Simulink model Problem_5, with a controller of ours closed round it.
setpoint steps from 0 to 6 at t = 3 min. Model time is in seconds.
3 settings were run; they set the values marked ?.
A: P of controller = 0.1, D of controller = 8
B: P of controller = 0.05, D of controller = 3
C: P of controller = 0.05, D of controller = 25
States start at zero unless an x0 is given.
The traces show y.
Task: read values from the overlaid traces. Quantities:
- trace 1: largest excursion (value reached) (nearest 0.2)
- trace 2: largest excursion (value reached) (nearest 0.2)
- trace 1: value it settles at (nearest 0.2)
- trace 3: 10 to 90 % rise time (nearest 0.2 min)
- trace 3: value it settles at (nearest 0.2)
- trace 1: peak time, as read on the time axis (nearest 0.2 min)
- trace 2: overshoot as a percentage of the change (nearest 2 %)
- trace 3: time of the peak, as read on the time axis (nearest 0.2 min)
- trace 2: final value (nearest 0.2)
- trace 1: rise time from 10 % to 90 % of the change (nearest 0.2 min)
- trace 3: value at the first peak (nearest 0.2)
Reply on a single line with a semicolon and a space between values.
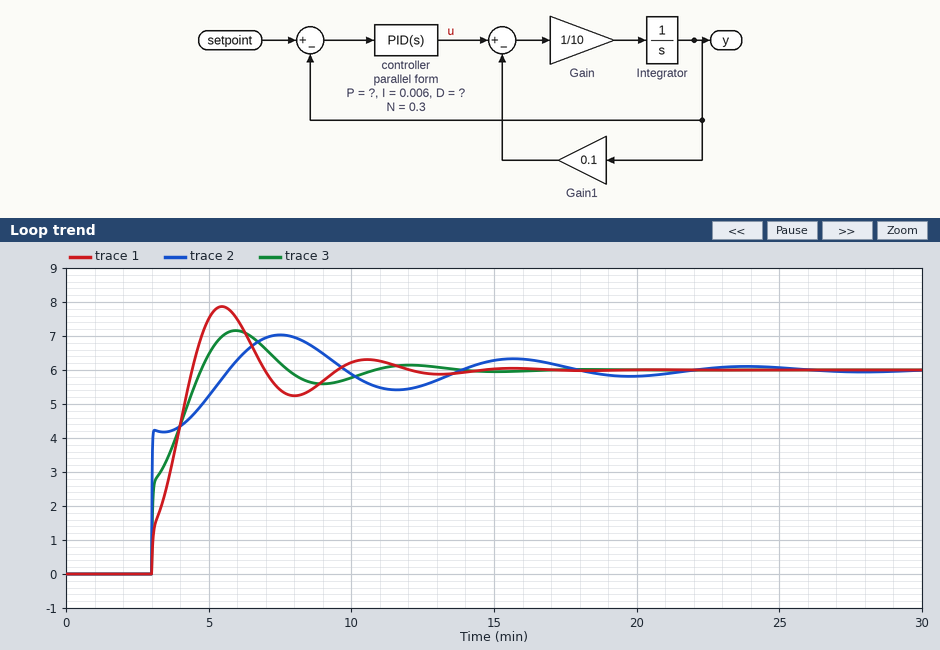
7.8; 7.0; 6.0; 1.4 min; 6.0; 5.4 min; 18 %; 6.0 min; 6.0; 1.2 min; 7.2
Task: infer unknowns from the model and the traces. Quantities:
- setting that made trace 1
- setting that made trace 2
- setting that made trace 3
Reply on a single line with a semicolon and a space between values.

B; C; A
